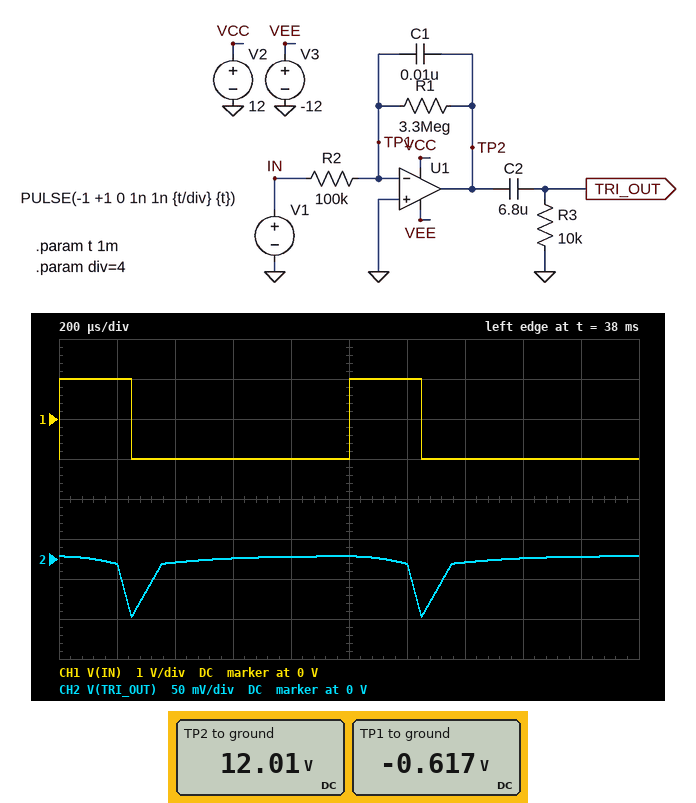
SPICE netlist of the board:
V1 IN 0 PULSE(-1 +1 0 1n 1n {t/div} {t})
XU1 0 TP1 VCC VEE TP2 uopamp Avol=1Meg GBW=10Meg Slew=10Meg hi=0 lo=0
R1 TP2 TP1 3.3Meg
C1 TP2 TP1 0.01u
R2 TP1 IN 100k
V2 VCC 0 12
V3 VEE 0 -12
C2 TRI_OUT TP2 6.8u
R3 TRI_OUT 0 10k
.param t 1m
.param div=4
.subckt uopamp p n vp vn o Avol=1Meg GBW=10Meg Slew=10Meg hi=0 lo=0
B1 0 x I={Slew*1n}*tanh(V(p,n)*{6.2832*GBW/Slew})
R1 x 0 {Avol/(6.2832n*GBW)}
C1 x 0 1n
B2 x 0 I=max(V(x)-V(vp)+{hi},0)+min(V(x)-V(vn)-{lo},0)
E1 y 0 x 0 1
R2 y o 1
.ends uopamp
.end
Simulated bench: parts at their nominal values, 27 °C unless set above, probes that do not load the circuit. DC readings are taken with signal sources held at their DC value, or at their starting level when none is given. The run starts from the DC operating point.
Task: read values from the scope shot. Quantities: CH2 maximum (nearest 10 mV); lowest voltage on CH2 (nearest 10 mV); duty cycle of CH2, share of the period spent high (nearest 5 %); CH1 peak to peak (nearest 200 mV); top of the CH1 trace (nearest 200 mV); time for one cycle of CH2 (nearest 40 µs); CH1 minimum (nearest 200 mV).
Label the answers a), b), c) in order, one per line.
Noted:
a) 0 V
b) -70 mV
c) 90 %
d) 2.0 V
e) 1.0 V
f) 1.00 ms
g) -1.0 V
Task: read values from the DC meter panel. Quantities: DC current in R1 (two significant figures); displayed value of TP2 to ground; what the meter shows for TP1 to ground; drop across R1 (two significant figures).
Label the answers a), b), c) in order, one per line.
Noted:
a) 3.8 µA
b) 12.01 V
c) -0.617 V
d) 13 V
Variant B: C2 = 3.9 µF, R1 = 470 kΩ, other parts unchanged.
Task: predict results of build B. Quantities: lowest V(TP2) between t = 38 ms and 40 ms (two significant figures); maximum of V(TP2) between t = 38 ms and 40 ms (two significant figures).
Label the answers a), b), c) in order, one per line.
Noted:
a) 2.2 V
b) 2.5 V
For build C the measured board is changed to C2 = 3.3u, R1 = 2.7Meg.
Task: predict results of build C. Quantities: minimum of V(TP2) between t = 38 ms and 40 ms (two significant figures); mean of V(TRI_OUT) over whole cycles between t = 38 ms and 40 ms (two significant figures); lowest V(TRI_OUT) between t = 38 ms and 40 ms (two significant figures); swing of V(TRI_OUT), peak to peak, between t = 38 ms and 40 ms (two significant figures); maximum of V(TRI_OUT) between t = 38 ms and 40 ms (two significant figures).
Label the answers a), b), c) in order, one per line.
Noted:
a) 12 V
b) -15 mV
c) -160 mV
d) 190 mV
e) 29 mV
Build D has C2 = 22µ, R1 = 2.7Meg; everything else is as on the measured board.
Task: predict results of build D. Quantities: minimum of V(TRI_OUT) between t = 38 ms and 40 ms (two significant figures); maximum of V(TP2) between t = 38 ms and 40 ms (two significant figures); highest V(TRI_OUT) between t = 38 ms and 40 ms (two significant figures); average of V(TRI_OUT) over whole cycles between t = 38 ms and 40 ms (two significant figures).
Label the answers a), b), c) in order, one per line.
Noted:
a) -180 mV
b) 12 V
c) 5.4 mV
d) -39 mV
